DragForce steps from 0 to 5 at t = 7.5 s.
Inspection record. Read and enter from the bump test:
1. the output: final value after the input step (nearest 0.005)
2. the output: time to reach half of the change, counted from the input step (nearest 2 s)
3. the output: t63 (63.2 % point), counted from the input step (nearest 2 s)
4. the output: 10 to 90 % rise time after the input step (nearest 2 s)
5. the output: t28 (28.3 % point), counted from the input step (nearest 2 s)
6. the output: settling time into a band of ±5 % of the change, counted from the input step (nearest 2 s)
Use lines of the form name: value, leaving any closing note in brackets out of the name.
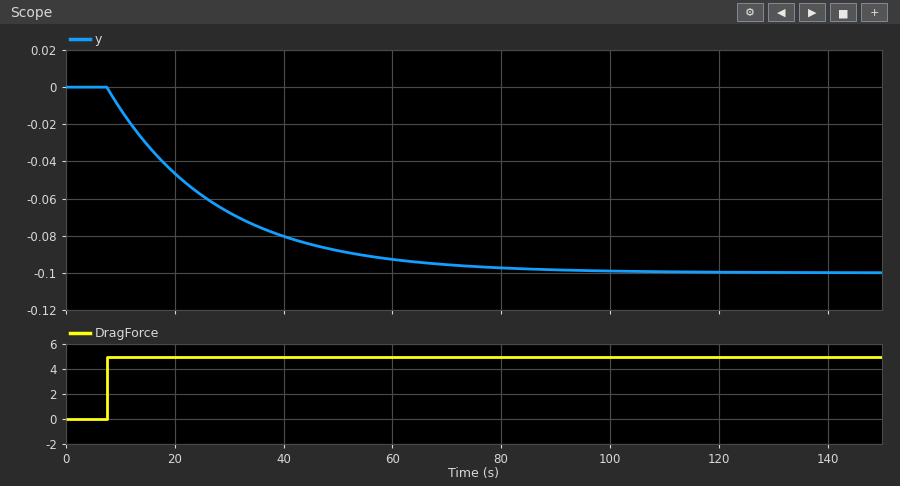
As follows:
the output: final value after the input step: -0.100
the output: time to reach half of the change, counted from the input step: 14 s
the output: t63 (63.2 % point), counted from the input step: 20 s
the output: 10 to 90 % rise time after the input step: 44 s
the output: t28 (28.3 % point), counted from the input step: 6 s
the output: settling time into a band of ±5 % of the change, counted from the input step: 60 s
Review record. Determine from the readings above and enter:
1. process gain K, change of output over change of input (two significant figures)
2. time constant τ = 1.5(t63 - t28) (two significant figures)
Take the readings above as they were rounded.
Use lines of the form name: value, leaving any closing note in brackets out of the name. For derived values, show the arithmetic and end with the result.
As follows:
process gain K, change of output over change of input: (-0.1 - 0) / 5 = -0.020
time constant τ = 1.5(t63 - t28): 1.5 × (20 - 6) = 21 s
